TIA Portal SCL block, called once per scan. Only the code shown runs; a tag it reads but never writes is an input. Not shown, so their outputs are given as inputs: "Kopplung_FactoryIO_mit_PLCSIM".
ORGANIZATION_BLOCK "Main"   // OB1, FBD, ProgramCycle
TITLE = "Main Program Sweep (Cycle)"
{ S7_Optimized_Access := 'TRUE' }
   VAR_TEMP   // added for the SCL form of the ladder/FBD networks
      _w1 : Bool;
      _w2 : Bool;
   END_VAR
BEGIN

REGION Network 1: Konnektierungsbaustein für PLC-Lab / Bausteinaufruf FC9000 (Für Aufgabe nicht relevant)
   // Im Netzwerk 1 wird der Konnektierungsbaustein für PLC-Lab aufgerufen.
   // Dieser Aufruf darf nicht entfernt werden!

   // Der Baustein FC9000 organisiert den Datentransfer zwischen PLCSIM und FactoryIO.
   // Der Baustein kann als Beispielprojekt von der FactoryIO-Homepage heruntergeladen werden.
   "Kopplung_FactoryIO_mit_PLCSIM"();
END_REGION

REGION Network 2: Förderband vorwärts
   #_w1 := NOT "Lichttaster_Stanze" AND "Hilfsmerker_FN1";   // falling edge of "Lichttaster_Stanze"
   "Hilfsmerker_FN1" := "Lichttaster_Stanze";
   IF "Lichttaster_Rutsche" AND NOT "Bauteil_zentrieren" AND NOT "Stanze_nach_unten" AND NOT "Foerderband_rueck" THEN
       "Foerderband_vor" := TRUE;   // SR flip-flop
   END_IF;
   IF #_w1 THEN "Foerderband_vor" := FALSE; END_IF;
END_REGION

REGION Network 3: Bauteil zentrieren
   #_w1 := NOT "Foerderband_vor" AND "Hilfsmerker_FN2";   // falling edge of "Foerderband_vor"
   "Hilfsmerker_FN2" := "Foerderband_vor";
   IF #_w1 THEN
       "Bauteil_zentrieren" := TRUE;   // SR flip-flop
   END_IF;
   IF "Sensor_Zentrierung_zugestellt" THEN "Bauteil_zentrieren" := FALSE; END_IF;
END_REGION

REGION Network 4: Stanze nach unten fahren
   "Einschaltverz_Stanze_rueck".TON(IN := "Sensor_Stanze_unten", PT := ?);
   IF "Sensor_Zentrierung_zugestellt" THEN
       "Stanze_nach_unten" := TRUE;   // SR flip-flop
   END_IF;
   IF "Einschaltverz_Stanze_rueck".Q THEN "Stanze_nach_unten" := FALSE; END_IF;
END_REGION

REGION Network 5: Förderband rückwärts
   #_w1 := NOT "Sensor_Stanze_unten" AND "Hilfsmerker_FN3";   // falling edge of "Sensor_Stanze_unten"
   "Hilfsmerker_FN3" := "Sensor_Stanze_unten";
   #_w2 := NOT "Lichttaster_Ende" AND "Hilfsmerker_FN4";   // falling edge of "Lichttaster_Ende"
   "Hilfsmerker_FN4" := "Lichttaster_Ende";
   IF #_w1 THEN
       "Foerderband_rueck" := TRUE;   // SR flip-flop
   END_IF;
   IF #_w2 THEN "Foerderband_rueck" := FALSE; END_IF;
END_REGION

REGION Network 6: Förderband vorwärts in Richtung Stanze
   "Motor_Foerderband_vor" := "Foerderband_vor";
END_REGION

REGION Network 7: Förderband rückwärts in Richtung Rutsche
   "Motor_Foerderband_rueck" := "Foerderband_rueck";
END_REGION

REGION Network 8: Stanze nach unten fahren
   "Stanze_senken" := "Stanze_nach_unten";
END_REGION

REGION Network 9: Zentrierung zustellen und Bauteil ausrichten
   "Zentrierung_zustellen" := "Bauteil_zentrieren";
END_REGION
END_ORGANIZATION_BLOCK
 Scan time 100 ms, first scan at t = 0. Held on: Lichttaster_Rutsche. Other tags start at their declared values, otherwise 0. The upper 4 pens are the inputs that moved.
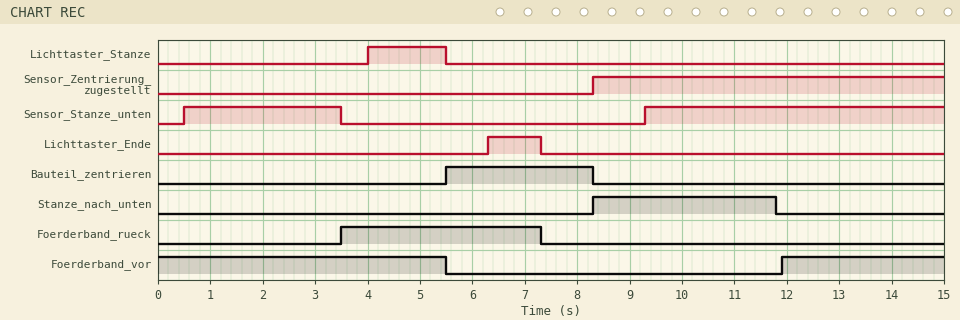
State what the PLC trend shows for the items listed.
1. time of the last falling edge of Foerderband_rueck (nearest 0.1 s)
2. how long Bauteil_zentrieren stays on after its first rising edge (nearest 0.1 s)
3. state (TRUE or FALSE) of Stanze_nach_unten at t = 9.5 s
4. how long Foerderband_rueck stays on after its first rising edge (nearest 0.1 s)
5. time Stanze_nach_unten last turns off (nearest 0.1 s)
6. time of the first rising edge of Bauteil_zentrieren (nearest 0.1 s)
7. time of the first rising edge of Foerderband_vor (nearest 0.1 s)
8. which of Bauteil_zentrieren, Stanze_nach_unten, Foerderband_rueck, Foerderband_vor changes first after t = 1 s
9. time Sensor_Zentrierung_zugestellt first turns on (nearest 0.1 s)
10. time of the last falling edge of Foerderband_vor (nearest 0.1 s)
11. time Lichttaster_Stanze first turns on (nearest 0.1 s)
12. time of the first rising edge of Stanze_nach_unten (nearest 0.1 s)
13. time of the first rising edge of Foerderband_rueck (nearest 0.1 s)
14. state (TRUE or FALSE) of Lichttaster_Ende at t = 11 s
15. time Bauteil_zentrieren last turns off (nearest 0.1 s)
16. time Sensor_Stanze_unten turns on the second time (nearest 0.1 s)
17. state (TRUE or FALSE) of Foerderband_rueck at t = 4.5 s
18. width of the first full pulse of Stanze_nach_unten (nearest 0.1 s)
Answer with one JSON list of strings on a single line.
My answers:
["7.3 s", "2.8 s", "TRUE", "3.8 s", "11.8 s", "5.5 s", "11.9 s", "Foerderband_rueck", "8.3 s", "5.5 s", "4.0 s", "8.3 s", "3.5 s", "FALSE", "8.3 s", "9.3 s", "TRUE", "3.5 s"]
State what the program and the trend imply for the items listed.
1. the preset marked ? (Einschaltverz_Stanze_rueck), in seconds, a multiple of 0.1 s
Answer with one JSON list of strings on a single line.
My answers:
["2.5 s"]
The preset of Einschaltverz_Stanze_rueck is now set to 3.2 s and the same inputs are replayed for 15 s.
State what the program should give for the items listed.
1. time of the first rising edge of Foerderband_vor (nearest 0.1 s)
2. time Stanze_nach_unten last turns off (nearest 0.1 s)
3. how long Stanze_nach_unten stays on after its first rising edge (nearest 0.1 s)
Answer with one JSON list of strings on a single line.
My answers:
["12.6 s", "12.5 s", "4.2 s"]
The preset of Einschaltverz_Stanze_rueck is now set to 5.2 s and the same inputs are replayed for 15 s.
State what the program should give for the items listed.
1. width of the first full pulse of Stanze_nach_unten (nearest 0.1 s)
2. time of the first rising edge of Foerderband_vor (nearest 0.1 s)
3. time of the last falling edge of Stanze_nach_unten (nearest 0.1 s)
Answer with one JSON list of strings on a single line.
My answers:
["6.2 s", "14.6 s", "14.5 s"]
